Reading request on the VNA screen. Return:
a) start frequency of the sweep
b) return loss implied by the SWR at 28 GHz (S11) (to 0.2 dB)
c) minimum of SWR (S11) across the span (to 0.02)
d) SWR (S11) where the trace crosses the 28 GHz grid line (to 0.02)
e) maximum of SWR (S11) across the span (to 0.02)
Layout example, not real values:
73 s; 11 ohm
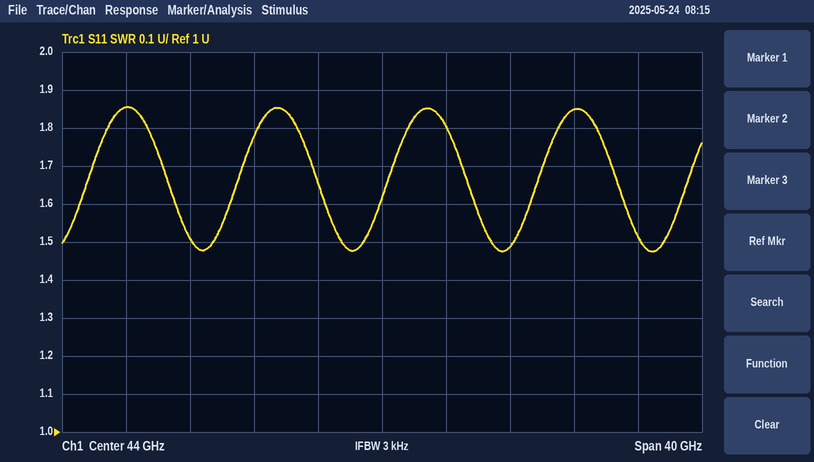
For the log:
24 GHz; 10.4 dB; 1.48; 1.86; 1.86
